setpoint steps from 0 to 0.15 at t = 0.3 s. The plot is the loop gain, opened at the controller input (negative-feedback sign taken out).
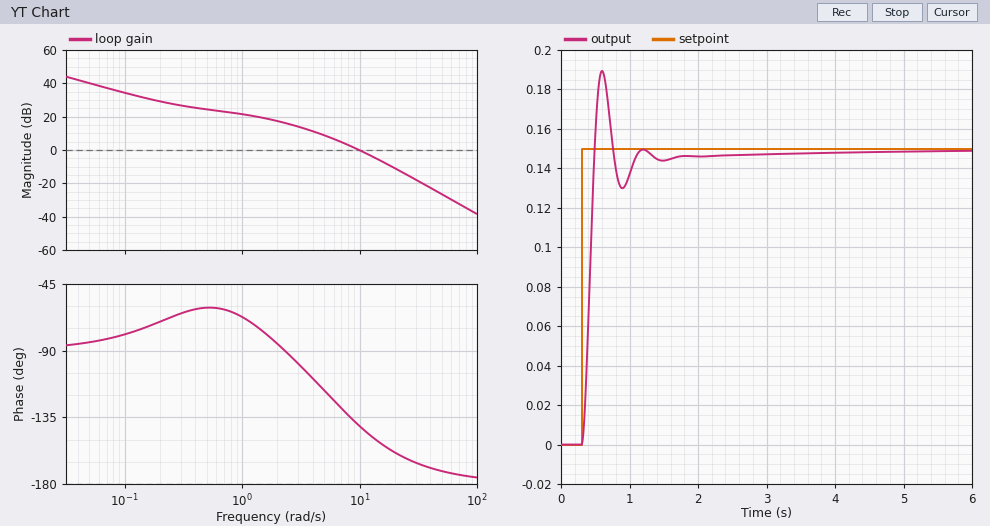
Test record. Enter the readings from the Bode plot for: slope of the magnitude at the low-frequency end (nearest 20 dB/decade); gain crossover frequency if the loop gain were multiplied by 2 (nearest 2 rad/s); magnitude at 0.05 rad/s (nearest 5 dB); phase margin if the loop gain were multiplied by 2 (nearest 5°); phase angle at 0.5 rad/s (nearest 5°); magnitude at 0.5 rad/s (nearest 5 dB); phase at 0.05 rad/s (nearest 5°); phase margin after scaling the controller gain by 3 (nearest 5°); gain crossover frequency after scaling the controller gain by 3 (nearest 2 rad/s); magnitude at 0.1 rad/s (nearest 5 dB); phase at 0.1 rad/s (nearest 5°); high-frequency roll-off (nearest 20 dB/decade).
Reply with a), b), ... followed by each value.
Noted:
a) -20 dB/decade
b) 14 rad/s
c) 40 dB
d) 30°
e) -60°
f) 25 dB
g) -85°
h) 25°
i) 18 rad/s
j) 35 dB
k) -80°
l) -40 dB/decade
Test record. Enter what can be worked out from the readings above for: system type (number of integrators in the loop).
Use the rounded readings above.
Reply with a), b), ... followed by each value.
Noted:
a) 1
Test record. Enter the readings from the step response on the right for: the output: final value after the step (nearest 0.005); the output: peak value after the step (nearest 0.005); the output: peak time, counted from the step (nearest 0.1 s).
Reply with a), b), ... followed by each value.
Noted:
a) 0.150
b) 0.190
c) 0.3 s
